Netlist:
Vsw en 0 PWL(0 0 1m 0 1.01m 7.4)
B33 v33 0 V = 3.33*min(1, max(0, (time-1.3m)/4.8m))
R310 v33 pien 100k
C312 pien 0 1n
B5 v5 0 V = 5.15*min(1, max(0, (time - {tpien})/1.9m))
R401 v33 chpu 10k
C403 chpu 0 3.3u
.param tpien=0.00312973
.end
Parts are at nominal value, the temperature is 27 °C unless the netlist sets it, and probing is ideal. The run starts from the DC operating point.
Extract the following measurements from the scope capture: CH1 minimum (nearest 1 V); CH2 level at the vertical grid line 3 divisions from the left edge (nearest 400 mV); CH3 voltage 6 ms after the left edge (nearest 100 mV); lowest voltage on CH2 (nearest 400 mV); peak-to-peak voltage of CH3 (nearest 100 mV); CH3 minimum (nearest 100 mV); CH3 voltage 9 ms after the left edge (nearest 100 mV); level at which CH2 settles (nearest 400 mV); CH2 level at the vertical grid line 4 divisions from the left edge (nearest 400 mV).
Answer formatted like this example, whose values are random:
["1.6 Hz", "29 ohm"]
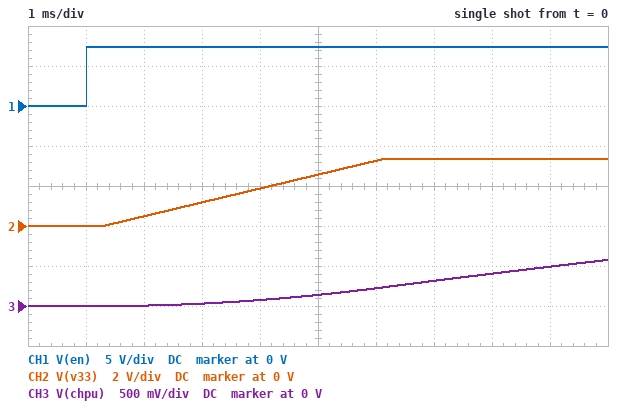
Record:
["0 V", "1.2 V", "200 mV", "0 V", "600 mV", "0 V", "500 mV", "3.2 V", "2.0 V"]
